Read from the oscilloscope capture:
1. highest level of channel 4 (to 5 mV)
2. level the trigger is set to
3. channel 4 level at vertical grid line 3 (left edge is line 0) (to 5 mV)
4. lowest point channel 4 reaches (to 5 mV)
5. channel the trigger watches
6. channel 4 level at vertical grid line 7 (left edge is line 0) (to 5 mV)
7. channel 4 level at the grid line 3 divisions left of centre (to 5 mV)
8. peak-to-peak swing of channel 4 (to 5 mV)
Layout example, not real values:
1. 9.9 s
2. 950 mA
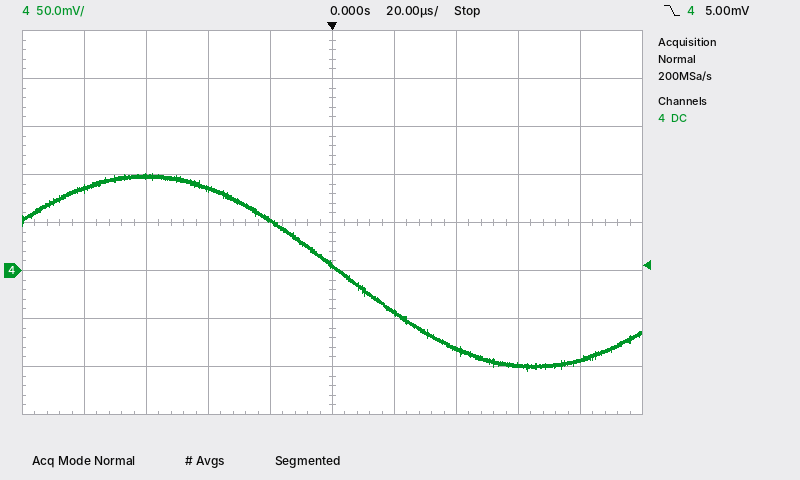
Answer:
1. 100 mV
2. 5.00 mV
3. 85 mV
4. -105 mV
5. channel 4
6. -80 mV
7. 100 mV
8. 205 mV
